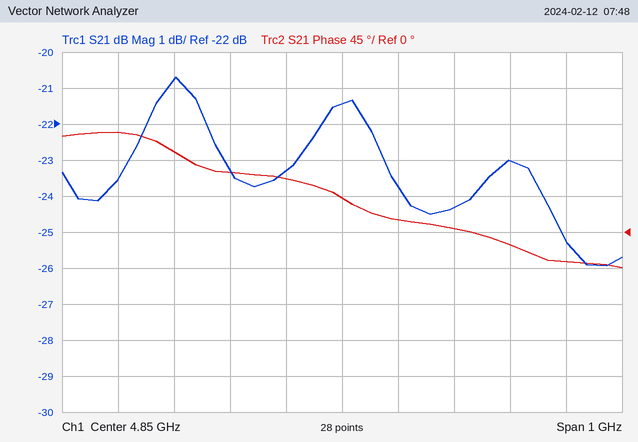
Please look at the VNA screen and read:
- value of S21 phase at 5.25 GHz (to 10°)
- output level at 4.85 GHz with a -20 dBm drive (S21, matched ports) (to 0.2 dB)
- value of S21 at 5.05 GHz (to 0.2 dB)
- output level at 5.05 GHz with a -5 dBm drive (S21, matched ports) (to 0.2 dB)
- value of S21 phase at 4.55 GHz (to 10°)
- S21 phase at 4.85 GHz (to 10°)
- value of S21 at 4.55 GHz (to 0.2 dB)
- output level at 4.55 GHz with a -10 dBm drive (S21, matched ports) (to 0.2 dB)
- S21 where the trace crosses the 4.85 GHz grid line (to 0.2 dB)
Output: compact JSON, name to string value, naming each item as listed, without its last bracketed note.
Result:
{"value of S21 phase at 5.25 GHz": "-40°", "output level at 4.85 GHz with a -20 dBm drive (S21, matched ports)": "-41.4 dBm", "value of S21 at 5.05 GHz": "-24.4 dB", "output level at 5.05 GHz with a -5 dBm drive (S21, matched ports)": "-29.4 dBm", "value of S21 phase at 4.55 GHz": "100°", "S21 phase at 4.85 GHz": "40°", "value of S21 at 4.55 GHz": "-20.8 dB", "output level at 4.55 GHz with a -10 dBm drive (S21, matched ports)": "-30.8 dBm", "S21 where the trace crosses the 4.85 GHz grid line": "-21.4 dB"}
